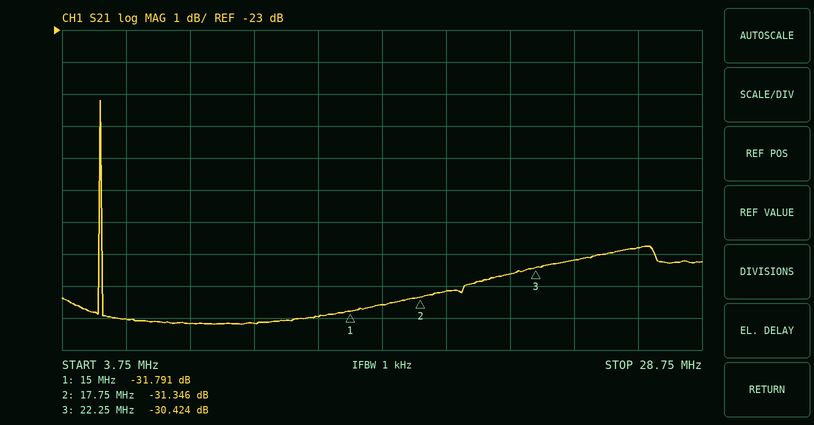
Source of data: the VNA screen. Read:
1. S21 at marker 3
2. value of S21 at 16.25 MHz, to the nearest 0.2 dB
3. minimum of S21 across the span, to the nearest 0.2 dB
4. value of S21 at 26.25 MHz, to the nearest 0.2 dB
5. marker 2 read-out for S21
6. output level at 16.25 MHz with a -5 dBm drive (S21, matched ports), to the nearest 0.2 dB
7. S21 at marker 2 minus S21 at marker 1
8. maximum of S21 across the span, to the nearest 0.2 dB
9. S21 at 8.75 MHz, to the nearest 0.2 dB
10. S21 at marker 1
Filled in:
-30.424 dB
-31.6 dB
-32.2 dB
-29.8 dB
-31.346 dB
-36.6 dBm
0.445 dB
-25.2 dB
-32.2 dB
-31.791 dB
